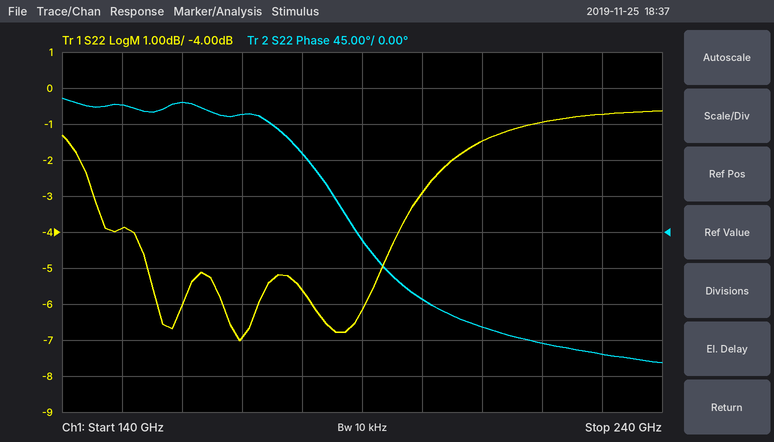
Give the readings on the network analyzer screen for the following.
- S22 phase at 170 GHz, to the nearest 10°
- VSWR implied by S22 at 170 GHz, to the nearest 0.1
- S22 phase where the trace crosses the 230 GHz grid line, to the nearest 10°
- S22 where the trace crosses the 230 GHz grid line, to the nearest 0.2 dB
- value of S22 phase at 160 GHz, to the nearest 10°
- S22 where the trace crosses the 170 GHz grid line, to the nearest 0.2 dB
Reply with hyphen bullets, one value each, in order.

- 150°
- 2.6
- -150°
- -0.8 dB
- 160°
- -7.0 dB
